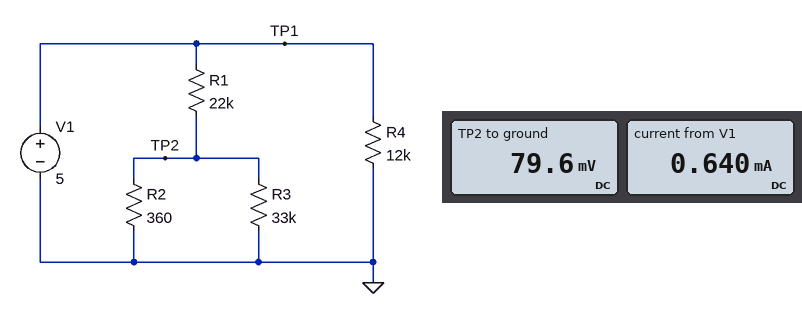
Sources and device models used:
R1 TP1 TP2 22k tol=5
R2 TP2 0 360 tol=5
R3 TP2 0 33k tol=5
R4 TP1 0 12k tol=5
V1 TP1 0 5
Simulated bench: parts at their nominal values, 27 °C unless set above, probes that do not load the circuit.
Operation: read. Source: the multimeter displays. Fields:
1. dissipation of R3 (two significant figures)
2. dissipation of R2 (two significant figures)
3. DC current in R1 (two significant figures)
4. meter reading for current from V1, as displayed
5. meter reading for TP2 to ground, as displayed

190 nW
18 µW
220 µA
0.640 mA
79.6 mV
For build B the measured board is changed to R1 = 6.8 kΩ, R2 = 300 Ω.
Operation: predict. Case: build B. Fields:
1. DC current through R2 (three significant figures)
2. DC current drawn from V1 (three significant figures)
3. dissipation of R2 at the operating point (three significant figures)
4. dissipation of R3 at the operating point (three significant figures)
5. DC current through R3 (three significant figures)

698 µA
1.12 mA
146 µW
1.33 µW
6.35 µA
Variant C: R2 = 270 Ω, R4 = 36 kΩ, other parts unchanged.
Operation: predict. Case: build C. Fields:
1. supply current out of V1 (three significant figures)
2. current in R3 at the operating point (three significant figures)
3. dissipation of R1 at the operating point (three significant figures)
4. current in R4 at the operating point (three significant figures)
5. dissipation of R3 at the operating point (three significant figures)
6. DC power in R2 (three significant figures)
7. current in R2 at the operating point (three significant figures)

363 µA
1.82 µA
1.11 mW
139 µA
110 nW
13.4 µW
223 µA
